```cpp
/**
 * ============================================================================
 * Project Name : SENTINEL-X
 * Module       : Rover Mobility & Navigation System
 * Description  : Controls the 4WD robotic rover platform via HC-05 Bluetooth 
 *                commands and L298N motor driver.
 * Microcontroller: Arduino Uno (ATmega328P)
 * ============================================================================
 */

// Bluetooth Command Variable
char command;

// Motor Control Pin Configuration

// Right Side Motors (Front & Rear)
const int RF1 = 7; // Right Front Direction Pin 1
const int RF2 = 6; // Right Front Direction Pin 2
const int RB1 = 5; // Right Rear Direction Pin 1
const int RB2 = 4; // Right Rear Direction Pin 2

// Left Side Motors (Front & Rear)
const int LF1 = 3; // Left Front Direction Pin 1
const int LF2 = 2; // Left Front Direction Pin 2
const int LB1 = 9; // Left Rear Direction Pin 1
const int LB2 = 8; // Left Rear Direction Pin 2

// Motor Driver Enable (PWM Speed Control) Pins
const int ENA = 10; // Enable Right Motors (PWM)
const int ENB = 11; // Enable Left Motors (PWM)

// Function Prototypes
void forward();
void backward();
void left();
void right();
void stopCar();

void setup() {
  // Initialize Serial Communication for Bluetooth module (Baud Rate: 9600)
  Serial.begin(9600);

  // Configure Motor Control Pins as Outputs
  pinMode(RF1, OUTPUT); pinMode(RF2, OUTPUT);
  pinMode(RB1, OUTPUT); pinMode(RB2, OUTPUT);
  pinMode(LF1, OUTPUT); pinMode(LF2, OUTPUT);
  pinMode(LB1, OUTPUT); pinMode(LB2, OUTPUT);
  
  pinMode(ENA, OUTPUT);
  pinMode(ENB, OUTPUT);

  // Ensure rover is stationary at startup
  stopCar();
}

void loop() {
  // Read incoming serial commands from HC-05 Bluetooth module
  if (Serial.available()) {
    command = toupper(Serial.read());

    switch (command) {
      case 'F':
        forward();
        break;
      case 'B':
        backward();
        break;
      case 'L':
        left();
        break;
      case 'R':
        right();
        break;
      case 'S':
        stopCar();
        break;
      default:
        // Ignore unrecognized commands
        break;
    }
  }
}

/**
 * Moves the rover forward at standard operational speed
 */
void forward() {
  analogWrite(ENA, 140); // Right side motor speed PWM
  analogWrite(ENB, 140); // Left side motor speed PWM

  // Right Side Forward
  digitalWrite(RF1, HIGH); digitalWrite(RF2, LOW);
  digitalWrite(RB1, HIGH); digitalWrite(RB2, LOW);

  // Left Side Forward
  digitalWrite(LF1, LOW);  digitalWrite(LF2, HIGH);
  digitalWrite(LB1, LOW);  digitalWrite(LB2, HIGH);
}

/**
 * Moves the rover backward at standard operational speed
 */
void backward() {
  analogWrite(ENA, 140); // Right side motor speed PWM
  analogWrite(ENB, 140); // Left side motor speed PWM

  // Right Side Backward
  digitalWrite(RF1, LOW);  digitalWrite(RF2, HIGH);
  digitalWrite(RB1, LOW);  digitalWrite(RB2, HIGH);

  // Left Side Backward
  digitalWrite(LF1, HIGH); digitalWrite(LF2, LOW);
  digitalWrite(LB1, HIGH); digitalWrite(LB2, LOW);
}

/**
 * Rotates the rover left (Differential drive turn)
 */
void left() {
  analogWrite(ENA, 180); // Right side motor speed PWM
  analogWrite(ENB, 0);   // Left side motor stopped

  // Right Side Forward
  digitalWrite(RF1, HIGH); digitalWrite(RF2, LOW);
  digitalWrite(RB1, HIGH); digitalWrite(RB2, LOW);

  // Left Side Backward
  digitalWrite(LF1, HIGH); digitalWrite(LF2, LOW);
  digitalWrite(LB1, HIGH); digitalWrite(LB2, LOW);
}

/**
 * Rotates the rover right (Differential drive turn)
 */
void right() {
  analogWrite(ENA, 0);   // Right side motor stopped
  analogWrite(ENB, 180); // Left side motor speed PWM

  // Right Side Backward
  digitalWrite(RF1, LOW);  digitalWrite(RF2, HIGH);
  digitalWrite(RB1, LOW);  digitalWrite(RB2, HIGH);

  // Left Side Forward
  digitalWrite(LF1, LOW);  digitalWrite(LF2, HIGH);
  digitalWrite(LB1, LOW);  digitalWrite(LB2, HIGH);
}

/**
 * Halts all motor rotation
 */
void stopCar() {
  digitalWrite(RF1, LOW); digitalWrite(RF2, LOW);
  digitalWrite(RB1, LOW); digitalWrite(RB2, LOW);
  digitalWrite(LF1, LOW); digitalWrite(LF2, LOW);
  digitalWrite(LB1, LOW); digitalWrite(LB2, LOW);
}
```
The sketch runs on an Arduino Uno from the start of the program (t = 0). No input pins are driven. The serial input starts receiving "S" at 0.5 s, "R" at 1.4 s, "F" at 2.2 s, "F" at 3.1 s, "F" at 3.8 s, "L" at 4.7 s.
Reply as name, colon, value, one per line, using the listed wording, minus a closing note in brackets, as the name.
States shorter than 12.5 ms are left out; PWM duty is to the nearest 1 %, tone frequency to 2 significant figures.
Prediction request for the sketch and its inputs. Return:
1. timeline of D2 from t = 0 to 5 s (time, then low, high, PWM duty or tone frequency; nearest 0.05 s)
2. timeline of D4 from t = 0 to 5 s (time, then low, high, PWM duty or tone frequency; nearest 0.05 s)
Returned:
timeline of D2 from t = 0 to 5 s: 0 s low; 1.4 s high; 4.7 s low
timeline of D4 from t = 0 to 5 s: 0 s low; 1.4 s high; 2.2 s low
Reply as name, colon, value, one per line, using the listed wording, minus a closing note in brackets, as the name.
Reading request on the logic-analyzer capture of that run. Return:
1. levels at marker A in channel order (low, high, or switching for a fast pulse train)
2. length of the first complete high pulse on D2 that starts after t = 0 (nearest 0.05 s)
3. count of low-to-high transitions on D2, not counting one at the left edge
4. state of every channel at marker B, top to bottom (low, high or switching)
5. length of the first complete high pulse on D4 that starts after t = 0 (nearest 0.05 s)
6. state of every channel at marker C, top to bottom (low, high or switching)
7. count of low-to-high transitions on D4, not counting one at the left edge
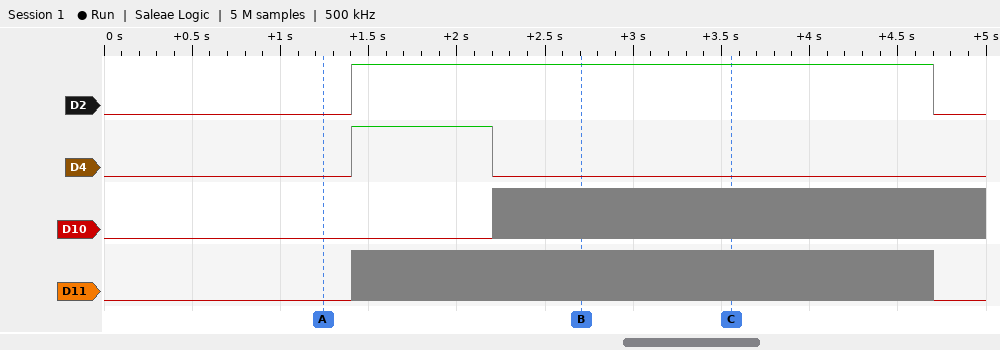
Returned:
levels at marker A in channel order: D2 low, D4 low, D10 low, D11 low
length of the first complete high pulse on D2 that starts after t = 0: 3.30 s
count of low-to-high transitions on D2, not counting one at the left edge: 1
state of every channel at marker B, top to bottom: D2 high, D4 low, D10 switching, D11 switching
length of the first complete high pulse on D4 that starts after t = 0: 0.80 s
state of every channel at marker C, top to bottom: D2 high, D4 low, D10 switching, D11 switching
count of low-to-high transitions on D4, not counting one at the left edge: 1
